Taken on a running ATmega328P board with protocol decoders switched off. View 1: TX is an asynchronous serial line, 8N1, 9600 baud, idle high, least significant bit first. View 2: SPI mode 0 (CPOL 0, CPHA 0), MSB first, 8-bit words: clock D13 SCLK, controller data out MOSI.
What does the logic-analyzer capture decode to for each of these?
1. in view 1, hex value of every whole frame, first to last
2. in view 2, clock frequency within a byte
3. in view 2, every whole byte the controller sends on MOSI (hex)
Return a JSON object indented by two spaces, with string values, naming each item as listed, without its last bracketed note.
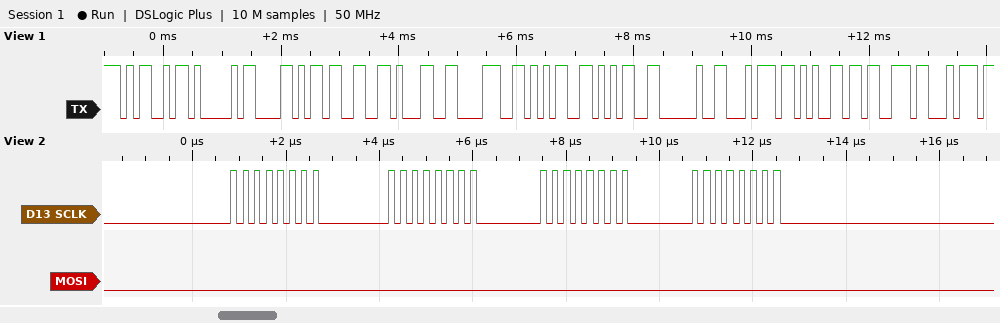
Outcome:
{
  "in view 1, hex value of every whole frame, first to last": "0x4D 0x41 0x58 0x33 0x31 0x38 0x35 0x35 0x20 0x74 0x65 0x73 0x74",
  "in view 2, clock frequency within a byte": "4 MHz",
  "in view 2, every whole byte the controller sends on MOSI": "00 00 00 00"
}
